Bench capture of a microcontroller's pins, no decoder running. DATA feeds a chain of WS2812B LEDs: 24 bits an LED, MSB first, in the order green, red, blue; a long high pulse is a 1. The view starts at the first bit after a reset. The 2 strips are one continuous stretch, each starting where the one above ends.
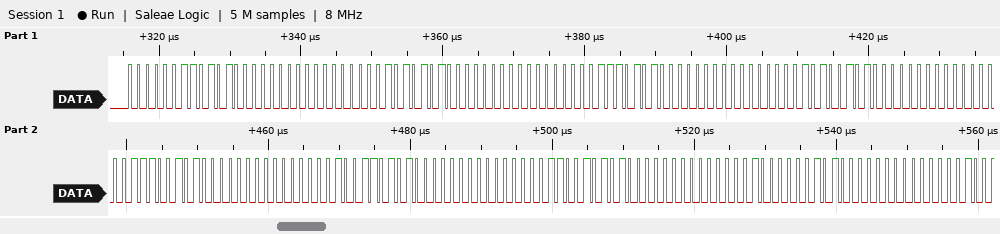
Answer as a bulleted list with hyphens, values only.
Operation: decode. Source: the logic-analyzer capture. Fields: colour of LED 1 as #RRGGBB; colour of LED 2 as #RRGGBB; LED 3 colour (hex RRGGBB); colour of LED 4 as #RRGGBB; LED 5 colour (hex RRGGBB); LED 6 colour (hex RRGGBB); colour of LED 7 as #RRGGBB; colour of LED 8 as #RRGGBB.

- #500300
- #500500
- #500700
- #500A00
- #500E00
- #501300
- #501900
- #502000
